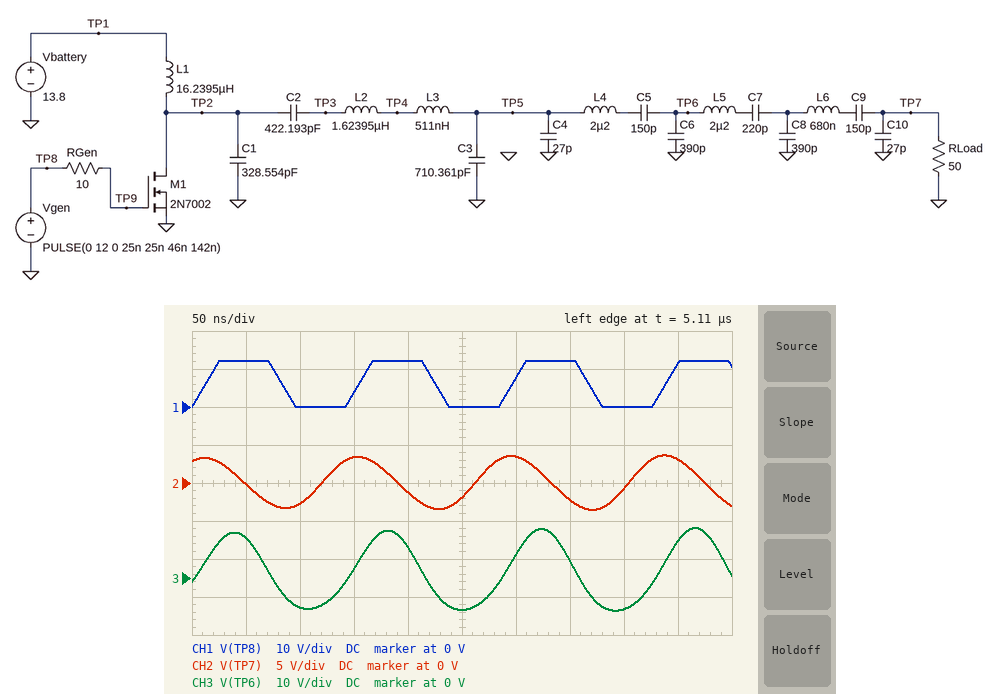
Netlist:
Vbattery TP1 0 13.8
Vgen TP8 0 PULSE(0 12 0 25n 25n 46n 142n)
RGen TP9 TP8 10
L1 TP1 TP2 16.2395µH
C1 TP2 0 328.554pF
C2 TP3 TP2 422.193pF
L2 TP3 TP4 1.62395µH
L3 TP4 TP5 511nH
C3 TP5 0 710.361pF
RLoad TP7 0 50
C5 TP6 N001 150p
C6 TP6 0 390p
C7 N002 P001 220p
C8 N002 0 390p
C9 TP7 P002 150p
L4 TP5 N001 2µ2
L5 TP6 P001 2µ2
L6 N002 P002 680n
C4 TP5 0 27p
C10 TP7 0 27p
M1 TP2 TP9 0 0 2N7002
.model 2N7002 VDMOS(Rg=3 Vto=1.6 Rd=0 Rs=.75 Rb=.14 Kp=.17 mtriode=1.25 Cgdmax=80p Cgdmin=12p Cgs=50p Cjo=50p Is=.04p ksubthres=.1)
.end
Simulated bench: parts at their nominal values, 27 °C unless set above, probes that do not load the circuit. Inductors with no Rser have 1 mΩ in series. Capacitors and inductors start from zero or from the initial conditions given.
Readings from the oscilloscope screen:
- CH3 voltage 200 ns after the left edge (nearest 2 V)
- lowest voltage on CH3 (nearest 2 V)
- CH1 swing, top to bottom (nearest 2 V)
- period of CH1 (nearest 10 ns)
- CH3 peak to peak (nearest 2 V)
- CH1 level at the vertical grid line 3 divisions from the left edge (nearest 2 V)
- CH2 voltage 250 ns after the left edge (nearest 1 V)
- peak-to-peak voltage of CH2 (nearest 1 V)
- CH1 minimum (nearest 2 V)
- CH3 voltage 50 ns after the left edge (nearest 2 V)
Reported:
8 V
-8 V
12 V
140 ns
22 V
4 V
-2 V
7 V
0 V
10 V
